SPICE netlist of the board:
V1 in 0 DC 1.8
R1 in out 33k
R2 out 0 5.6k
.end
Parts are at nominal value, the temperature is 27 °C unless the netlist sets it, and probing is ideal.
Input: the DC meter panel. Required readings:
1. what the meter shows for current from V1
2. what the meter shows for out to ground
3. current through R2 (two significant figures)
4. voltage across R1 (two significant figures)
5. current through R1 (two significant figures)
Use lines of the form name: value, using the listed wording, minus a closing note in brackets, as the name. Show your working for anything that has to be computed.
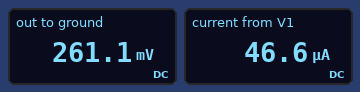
what the meter shows for current from V1: 46.6 µA
what the meter shows for out to ground: 261.1 mV
current through R2: (261.1 mV) / 5.6 kΩ = 47 µA
voltage across R1: 1.8 V - 261.1 mV = 1.5 V
current through R1: (1.8 V - 261.1 mV) / 33 kΩ = 47 µA
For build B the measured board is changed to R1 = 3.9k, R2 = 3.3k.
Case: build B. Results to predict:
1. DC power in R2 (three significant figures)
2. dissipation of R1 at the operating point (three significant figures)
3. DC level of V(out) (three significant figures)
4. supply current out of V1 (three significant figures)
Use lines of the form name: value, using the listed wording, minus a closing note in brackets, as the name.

DC power in R2: 206 µW
dissipation of R1 at the operating point: 244 µW
DC level of V(out): 825 mV
supply current out of V1: 250 µA
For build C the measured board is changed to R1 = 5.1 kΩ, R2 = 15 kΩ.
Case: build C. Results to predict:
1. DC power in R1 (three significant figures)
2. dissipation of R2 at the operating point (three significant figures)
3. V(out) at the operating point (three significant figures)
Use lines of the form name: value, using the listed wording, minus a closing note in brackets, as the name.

DC power in R1: 40.9 µW
dissipation of R2 at the operating point: 120 µW
V(out) at the operating point: 1.34 V
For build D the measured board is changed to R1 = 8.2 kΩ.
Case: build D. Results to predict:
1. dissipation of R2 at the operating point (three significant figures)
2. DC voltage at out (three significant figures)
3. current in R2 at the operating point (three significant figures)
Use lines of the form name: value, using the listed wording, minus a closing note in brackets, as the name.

dissipation of R2 at the operating point: 95.3 µW
DC voltage at out: 730 mV
current in R2 at the operating point: 130 µA
